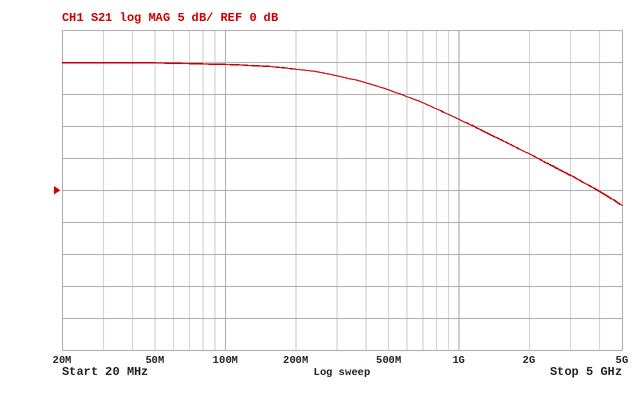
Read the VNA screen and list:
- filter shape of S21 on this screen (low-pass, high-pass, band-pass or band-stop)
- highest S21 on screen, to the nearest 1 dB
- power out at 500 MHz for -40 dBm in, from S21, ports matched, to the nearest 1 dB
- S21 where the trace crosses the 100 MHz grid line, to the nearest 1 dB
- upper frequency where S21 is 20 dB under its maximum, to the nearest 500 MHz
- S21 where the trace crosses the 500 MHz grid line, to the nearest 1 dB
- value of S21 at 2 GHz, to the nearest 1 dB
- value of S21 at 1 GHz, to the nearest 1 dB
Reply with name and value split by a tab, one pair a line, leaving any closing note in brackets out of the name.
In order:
filter shape of S21 on this screen	low-pass
highest S21 on screen, to the nearest 1 dB	20 dB
power out at 500 MHz for -40 dBm in, from S21, ports matched, to the nearest 1 dB	-24 dBm
S21 where the trace crosses the 100 MHz grid line, to the nearest 1 dB	20 dB
upper frequency where S21 is 20 dB under its maximum, to the nearest 500 MHz	4.0 GHz
S21 where the trace crosses the 500 MHz grid line, to the nearest 1 dB	16 dB
value of S21 at 2 GHz, to the nearest 1 dB	6 dB
value of S21 at 1 GHz, to the nearest 1 dB	11 dB
